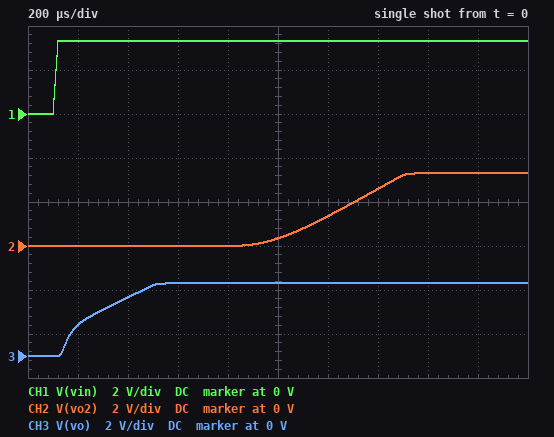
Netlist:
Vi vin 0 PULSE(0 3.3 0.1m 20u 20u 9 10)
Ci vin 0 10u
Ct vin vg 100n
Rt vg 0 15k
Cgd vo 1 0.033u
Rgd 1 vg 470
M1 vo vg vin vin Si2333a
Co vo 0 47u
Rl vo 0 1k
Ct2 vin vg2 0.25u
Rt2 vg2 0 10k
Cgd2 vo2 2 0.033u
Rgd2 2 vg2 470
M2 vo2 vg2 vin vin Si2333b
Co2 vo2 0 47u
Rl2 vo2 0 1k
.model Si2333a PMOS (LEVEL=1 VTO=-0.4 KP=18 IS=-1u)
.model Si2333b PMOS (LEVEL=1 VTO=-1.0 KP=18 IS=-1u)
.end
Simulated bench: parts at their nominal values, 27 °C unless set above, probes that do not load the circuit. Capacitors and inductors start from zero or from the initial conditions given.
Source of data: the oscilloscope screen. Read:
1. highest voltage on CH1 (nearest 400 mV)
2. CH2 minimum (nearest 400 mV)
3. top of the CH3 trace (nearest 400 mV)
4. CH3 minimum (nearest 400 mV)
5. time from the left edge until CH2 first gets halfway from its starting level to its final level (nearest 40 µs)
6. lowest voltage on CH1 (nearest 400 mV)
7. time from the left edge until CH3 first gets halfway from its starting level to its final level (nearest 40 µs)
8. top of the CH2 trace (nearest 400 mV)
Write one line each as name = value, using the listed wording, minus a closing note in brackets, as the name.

highest voltage on CH1 = 3.2 V
CH2 minimum = 0 V
top of the CH3 trace = 3.2 V
CH3 minimum = 0 V
time from the left edge until CH2 first gets halfway from its starting level to its final level = 1.24 ms
lowest voltage on CH1 = 0 V
time from the left edge until CH3 first gets halfway from its starting level to its final level = 240 µs
top of the CH2 trace = 3.2 V
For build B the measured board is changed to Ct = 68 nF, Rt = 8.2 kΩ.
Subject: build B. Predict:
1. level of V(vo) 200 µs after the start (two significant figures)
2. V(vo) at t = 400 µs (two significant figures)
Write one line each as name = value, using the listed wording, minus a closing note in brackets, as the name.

level of V(vo) 200 µs after the start = 2.4 V
V(vo) at t = 400 µs = 3.3 V
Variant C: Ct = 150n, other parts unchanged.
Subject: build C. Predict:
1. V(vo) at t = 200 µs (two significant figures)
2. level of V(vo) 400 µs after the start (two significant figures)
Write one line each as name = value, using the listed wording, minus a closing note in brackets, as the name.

V(vo) at t = 200 µs = 550 mV
level of V(vo) 400 µs after the start = 1.8 V
